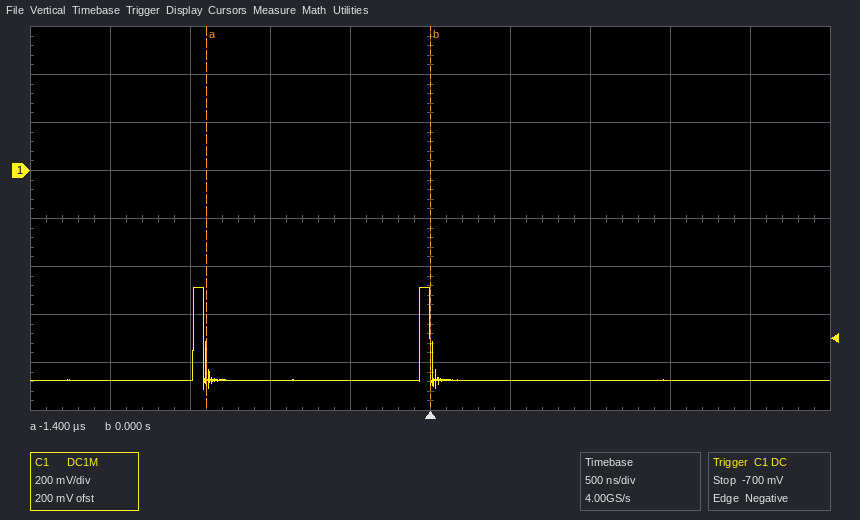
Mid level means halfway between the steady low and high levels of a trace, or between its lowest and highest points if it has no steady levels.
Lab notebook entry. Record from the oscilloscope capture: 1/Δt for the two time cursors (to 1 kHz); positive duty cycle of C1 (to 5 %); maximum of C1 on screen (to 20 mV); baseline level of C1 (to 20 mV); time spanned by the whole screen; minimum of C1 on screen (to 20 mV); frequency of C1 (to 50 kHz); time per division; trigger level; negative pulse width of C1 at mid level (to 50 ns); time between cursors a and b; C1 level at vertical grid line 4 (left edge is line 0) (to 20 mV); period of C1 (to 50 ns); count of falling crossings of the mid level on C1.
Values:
714 kHz
5 %
-480 mV
-880 mV
5 µs
-920 mV
700 kHz
500 ns
-700 mV
1.35 µs
1.40 µs
-880 mV
1.40 µs
2
